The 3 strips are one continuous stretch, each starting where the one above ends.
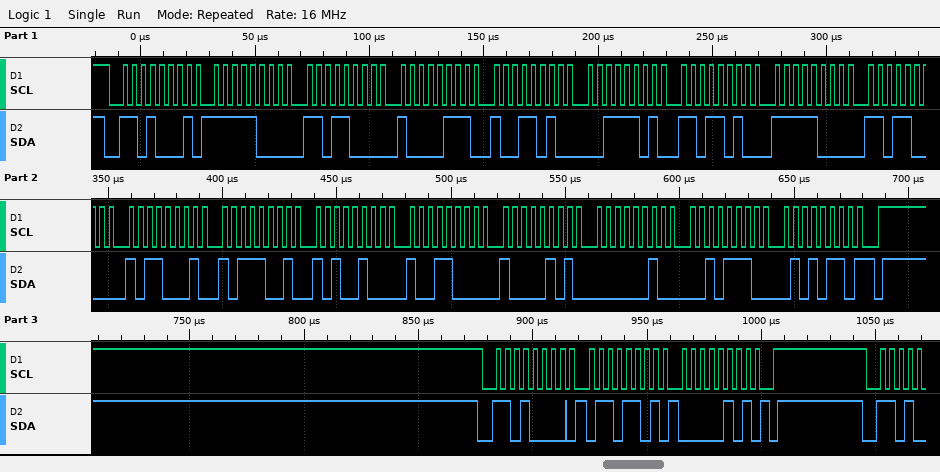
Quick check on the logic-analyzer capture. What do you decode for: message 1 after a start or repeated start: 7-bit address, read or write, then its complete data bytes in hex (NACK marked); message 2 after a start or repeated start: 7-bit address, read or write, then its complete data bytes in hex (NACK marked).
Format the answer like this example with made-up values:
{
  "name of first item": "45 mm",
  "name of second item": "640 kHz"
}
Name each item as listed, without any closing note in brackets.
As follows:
{
  "message 1 after a start or repeated start: 7-bit address, read or write, then its complete data bytes in hex": "0x68 read: F8 D8 87 9A 3D DA F8 D8 B1 B9 A4 98 85 02 2E 56 NACK",
  "message 2 after a start or repeated start: 7-bit address, read or write, then its complete data bytes in hex": "0x68 write: 6D 05"
}
